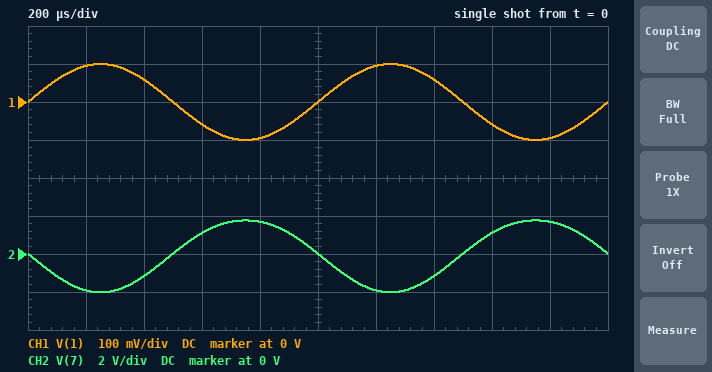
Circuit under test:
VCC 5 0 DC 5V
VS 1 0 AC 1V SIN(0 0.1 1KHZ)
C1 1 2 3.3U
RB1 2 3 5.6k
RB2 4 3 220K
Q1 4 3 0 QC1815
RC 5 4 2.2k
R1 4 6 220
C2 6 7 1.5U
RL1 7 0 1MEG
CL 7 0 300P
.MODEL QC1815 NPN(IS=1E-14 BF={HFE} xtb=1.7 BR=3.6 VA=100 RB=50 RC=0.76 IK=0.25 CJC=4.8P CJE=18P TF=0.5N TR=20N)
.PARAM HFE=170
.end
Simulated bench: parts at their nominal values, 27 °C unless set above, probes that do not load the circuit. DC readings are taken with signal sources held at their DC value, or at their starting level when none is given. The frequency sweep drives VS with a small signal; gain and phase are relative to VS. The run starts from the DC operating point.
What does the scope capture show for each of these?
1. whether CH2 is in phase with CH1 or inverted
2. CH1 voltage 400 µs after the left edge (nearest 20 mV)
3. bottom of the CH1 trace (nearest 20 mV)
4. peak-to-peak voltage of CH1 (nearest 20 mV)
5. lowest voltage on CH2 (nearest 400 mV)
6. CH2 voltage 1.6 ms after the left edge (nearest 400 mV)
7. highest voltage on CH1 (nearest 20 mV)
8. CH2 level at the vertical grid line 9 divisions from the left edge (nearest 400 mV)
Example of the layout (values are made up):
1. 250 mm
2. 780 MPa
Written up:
1. inverted
2. 60 mV
3. -100 mV
4. 200 mV
5. -2.0 V
6. 1.2 V
7. 100 mV
8. 1.6 V
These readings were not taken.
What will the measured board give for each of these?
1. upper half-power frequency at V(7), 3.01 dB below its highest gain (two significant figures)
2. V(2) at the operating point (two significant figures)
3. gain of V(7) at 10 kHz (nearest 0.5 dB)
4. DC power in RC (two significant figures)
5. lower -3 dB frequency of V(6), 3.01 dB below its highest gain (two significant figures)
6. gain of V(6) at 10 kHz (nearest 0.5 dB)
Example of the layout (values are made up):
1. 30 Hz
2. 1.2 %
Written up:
1. 220 kHz
2. 660 mV
3. 26.0 dB
4. 3.4 mW
5. 6.9 Hz
6. 26.0 dB
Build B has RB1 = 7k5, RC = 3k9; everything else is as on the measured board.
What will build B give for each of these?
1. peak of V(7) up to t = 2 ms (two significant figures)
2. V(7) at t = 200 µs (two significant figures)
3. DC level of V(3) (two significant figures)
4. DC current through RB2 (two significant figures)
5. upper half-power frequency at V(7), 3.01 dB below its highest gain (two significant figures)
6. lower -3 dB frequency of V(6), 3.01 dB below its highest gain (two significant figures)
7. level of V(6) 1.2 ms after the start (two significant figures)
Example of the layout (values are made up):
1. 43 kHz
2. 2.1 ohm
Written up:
1. 1.7 V
2. -1.6 V
3. 650 mV
4. 4.9 µA
5. 170 kHz
6. 5.4 Hz
7. 150 mV
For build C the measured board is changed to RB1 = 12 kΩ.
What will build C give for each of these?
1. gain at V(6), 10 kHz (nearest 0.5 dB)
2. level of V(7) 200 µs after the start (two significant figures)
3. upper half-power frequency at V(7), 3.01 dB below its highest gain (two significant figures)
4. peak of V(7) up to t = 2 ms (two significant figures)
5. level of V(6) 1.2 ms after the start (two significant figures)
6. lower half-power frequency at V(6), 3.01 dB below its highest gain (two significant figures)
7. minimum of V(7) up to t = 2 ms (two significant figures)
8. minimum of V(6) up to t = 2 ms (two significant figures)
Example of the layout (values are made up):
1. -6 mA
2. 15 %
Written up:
1. 20.0 dB
2. -970 mV
3. 220 kHz
4. 1.0 V
5. 1.3 V
6. 3.6 Hz
7. -1.0 V
8. 1.2 V
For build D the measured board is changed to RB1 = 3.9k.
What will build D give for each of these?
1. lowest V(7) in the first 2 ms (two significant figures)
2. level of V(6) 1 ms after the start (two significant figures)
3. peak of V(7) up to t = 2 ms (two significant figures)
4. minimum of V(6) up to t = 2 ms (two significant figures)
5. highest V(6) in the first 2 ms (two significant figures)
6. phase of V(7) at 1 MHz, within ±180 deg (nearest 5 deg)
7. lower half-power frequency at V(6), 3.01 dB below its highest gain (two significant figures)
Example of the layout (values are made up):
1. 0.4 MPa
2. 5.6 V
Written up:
1. -2.1 V
2. 2.3 V
3. 2.1 V
4. 130 mV
5. 4.4 V
6. 75 deg
7. 9.2 Hz
